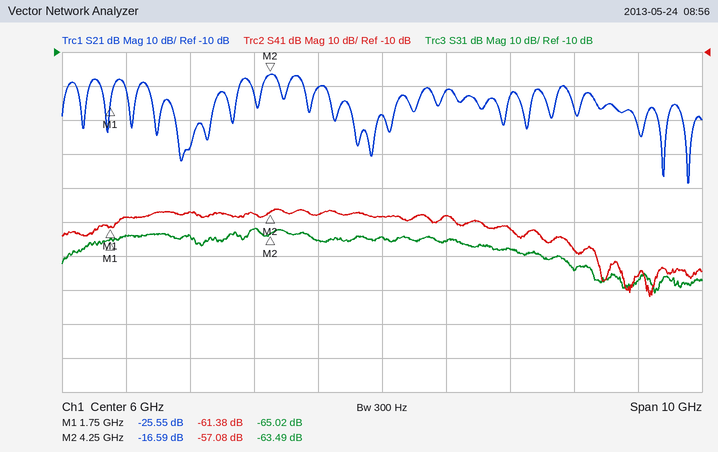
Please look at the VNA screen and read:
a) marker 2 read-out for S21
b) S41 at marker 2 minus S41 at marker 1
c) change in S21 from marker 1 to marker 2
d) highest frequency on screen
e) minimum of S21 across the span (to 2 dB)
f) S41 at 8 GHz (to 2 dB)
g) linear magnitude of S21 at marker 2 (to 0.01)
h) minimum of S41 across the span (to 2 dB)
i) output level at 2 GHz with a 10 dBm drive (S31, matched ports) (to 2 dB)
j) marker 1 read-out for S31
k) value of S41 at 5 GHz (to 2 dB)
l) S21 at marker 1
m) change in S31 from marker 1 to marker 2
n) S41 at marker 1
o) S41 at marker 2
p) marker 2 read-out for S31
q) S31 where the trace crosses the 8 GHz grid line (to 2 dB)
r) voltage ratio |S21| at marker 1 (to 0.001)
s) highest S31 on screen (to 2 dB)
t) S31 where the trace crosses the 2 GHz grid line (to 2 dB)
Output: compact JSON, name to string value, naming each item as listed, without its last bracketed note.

{"marker 2 read-out for S21": "-16.59 dB", "S41 at marker 2 minus S41 at marker 1": "4.30 dB", "change in S21 from marker 1 to marker 2": "8.96 dB", "highest frequency on screen": "11 GHz", "minimum of S21 across the span": "-48 dB", "S41 at 8 GHz": "-62 dB", "linear magnitude of S21 at marker 2": "0.15", "minimum of S41 across the span": "-82 dB", "output level at 2 GHz with a 10 dBm drive (S31, matched ports)": "-54 dBm", "marker 1 read-out for S31": "-65.02 dB", "value of S41 at 5 GHz": "-58 dB", "S21 at marker 1": "-25.55 dB", "change in S31 from marker 1 to marker 2": "1.53 dB", "S41 at marker 1": "-61.38 dB", "S41 at marker 2": "-57.08 dB", "marker 2 read-out for S31": "-63.49 dB", "S31 where the trace crosses the 8 GHz grid line": "-68 dB", "voltage ratio |S21| at marker 1": "0.053", "highest S31 on screen": "-62 dB", "S31 where the trace crosses the 2 GHz grid line": "-64 dB"}
